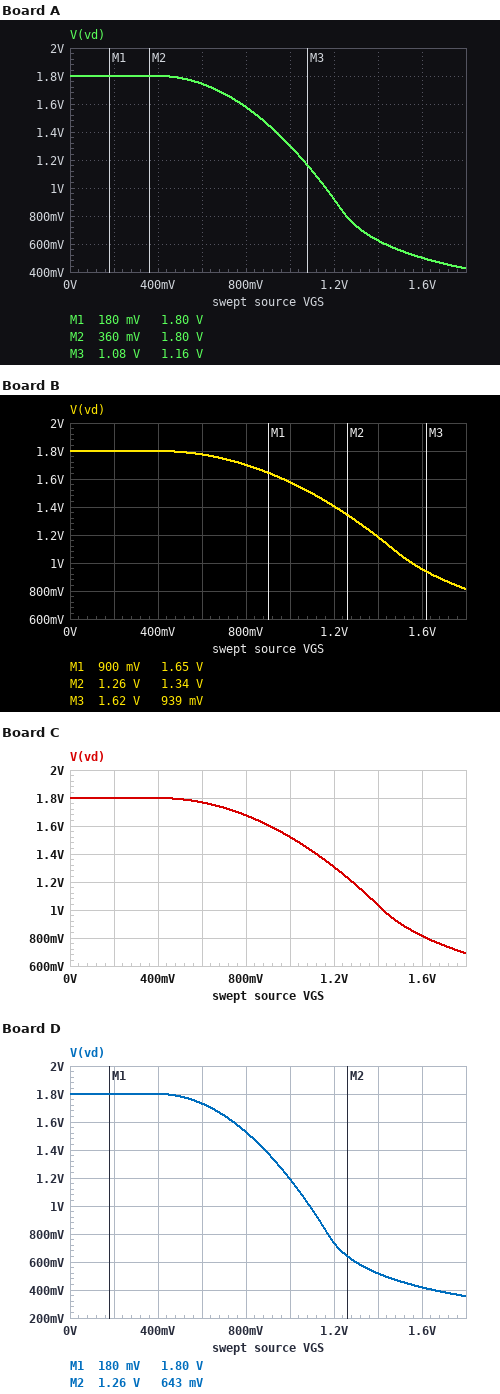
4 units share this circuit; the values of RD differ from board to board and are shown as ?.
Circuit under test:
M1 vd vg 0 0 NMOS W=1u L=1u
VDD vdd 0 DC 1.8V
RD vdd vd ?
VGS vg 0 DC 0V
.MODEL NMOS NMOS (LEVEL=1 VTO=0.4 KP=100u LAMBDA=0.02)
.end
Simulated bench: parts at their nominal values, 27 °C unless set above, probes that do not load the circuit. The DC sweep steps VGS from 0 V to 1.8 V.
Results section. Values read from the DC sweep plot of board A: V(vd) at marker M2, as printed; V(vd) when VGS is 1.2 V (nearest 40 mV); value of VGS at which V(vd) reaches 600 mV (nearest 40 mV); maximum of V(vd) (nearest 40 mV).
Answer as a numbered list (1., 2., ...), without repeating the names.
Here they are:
1. 1.80 V
2. 920 mV
3. 1.44 V
4. 1.80 V
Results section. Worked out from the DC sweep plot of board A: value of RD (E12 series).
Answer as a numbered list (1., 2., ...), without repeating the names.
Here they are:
1. 27 kΩ
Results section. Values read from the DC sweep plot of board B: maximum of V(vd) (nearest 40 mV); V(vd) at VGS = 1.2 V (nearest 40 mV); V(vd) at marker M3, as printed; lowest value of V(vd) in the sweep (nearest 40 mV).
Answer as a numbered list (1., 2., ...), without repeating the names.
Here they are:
1. 1.80 V
2. 1.40 V
3. 939 mV
4. 800 mV
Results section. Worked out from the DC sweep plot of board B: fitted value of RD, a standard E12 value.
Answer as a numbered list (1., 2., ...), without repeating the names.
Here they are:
1. 12 kΩ
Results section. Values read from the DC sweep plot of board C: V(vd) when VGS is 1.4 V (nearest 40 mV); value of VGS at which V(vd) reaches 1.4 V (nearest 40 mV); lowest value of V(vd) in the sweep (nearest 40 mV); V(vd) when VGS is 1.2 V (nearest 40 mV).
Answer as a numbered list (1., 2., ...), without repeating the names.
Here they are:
1. 1.04 V
2. 1.12 V
3. 680 mV
4. 1.32 V
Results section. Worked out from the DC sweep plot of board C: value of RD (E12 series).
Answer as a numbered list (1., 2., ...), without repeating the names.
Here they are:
1. 15 kΩ
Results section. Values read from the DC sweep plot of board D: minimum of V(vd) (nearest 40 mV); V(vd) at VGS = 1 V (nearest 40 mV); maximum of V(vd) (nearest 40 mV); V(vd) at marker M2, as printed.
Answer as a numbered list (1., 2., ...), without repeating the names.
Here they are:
1. 360 mV
2. 1.20 V
3. 1.80 V
4. 643 mV
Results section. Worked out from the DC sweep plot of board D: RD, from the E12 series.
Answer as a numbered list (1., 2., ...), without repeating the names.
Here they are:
1. 33 kΩ
